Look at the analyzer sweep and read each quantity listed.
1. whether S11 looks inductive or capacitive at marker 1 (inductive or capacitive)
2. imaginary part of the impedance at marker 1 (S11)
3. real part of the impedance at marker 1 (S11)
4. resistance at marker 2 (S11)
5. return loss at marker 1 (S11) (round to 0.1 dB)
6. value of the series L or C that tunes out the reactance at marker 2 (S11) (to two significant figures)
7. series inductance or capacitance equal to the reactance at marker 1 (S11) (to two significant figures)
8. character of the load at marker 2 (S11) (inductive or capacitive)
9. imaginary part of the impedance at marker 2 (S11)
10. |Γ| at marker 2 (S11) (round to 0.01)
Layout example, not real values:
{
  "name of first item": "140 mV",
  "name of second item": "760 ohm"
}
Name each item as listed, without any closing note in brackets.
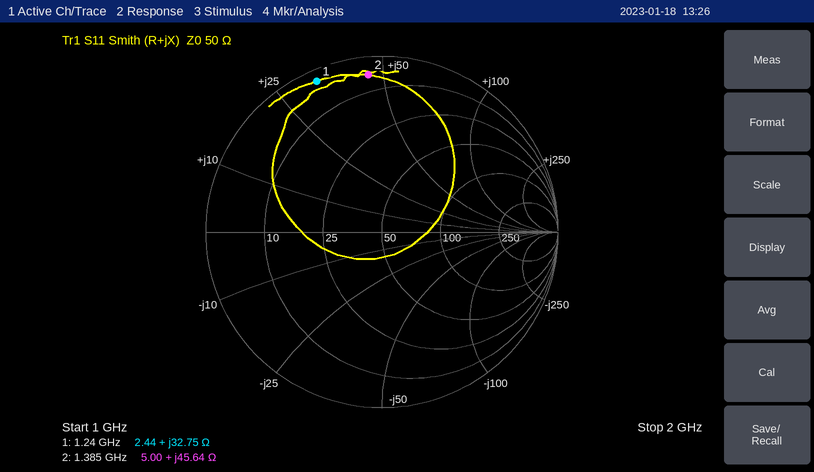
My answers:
{
  "whether S11 looks inductive or capacitive at marker 1": "inductive",
  "imaginary part of the impedance at marker 1": "+32.75 Ω",
  "real part of the impedance at marker 1": "2.44 Ω",
  "resistance at marker 2": "5.00 Ω",
  "return loss at marker 1 (S11)": "0.6 dB",
  "value of the series L or C that tunes out the reactance at marker 2 (S11)": "2.5 pF",
  "series inductance or capacitance equal to the reactance at marker 1 (S11)": "4.2 nH",
  "character of the load at marker 2 (S11)": "inductive",
  "imaginary part of the impedance at marker 2": "+45.64 Ω",
  "|Γ| at marker 2 (S11)": "0.90"
}
